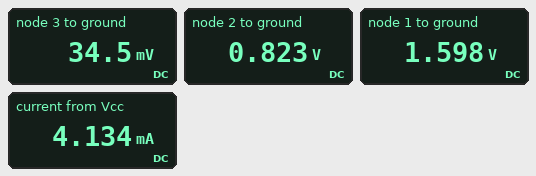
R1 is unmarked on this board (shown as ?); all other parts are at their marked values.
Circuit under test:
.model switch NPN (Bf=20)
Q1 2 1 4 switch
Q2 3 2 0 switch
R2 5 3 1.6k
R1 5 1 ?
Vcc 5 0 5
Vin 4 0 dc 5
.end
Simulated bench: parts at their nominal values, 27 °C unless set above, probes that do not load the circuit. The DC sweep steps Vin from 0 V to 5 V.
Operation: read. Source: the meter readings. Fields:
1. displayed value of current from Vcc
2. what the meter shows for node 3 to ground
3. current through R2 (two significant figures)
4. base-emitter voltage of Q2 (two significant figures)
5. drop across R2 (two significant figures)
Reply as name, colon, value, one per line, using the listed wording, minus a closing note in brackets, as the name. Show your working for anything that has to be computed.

displayed value of current from Vcc: 4.134 mA
what the meter shows for node 3 to ground: 34.5 mV
current through R2: (5 V - 34.5 mV) / 1.6 kΩ = 3.1 mA
base-emitter voltage of Q2: 823 mV = 820 mV
drop across R2: 5 V - 34.5 mV = 5.0 V
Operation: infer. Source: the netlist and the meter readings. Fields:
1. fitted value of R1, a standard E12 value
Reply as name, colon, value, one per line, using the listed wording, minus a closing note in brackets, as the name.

fitted value of R1, a standard E12 value: 3.3 kΩ
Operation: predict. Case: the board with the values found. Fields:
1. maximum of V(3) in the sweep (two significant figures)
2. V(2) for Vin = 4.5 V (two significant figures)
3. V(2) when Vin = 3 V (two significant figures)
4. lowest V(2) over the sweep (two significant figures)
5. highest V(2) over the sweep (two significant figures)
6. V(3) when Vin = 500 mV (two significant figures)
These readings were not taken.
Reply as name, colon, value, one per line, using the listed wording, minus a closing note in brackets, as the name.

maximum of V(3) in the sweep: 5.0 V
V(2) for Vin = 4.5 V: 820 mV
V(2) when Vin = 3 V: 820 mV
lowest V(2) over the sweep: 18 mV
highest V(2) over the sweep: 820 mV
V(3) when Vin = 500 mV: 5.0 V
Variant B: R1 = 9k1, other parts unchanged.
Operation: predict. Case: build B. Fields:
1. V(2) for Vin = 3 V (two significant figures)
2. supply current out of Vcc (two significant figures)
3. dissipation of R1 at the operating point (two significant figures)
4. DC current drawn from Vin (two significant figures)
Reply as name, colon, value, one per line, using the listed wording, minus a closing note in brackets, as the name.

V(2) for Vin = 3 V: 810 mV
supply current out of Vcc: 3.5 mA
dissipation of R1 at the operating point: 1.3 mW
DC current drawn from Vin: 380 µA
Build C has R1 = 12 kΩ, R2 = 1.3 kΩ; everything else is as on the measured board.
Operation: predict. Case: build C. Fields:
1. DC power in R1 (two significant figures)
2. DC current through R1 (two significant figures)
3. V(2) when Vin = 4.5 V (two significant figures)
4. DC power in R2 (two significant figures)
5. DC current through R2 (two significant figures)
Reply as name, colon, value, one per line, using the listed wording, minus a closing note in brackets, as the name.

DC power in R1: 990 µW
DC current through R1: 290 µA
V(2) when Vin = 4.5 V: 810 mV
DC power in R2: 19 mW
DC current through R2: 3.8 mA
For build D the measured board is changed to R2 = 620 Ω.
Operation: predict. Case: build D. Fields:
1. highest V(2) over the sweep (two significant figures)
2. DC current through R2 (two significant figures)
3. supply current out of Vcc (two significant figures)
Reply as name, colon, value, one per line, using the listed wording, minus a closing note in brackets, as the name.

highest V(2) over the sweep: 840 mV
DC current through R2: 8.0 mA
supply current out of Vcc: 9.0 mA
